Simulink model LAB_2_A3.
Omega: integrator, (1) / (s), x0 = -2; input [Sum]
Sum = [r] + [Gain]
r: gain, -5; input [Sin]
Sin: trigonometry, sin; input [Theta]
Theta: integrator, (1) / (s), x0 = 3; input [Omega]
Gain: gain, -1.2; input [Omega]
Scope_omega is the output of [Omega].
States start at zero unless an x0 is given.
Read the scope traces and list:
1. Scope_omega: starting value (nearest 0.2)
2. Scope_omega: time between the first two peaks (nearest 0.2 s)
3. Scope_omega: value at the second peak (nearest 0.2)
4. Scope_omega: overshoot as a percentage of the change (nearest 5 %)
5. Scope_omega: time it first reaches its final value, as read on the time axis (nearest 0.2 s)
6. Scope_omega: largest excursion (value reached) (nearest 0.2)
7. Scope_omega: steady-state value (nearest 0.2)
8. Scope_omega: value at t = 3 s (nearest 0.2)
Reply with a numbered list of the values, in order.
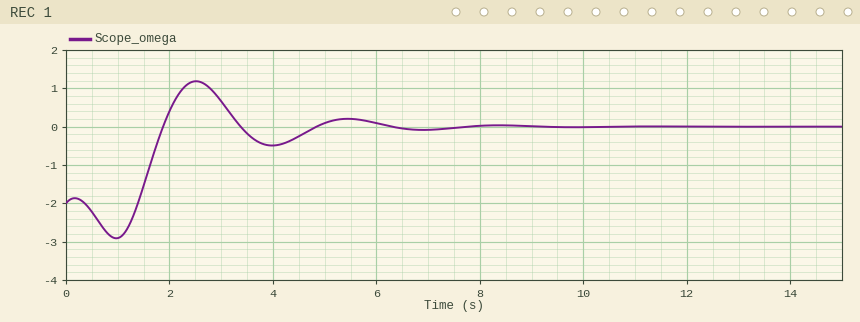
1. -2.0
2. 3.0 s
3. 0.2
4. 60 %
5. 1.8 s
6. 1.2
7. 0.0
8. 0.6
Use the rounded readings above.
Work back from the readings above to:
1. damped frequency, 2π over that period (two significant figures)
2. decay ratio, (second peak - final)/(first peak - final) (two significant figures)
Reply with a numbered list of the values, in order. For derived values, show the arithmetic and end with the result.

1. 2π / 3 = 2.1 rad/s
2. (0.2 - 0) / (1.2 - 0) = 0.17
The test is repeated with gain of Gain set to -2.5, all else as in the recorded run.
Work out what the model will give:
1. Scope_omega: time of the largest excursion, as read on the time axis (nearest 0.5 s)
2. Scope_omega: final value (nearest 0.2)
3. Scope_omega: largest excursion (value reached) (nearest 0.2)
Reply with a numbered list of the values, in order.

1. 3.0 s
2. 0.0
3. 0.2
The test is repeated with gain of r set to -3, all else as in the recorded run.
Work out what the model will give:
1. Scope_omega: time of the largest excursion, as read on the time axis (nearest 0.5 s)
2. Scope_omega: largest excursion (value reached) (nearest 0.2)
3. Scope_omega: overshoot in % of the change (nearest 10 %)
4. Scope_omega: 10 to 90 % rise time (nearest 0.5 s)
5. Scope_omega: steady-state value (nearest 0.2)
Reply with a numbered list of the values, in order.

1. 3.0 s
2. 0.6
3. 30 %
4. 2.0 s
5. 0.0
